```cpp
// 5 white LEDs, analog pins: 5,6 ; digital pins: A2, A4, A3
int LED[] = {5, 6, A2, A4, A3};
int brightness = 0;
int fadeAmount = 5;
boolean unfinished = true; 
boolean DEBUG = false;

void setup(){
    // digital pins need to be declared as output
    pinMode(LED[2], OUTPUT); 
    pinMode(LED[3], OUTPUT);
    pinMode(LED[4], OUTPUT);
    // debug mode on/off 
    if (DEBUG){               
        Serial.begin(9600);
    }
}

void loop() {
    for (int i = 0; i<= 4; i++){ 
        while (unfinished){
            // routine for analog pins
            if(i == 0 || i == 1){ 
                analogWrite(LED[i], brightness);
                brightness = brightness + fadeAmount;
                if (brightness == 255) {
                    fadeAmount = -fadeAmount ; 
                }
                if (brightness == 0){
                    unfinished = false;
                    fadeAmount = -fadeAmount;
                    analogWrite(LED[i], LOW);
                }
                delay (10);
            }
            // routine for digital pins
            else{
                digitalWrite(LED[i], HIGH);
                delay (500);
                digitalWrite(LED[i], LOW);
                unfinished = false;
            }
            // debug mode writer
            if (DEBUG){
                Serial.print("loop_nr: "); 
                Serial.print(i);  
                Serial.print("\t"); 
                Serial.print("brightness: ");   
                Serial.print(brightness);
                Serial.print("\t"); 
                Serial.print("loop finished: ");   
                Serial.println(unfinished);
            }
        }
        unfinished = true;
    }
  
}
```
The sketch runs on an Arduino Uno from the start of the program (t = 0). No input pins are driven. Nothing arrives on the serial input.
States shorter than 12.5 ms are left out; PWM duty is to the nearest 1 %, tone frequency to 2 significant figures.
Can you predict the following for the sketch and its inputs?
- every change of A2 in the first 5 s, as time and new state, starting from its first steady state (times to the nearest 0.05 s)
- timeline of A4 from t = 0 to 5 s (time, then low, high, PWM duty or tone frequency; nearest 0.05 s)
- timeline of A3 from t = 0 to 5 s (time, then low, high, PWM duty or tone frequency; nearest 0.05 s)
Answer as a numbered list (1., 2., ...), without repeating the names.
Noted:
1. 0 s low; 2.05 s high; 2.55 s low
2. 0 s low; 2.55 s high; 3.05 s low
3. 0 s low; 3.05 s high; 3.55 s low
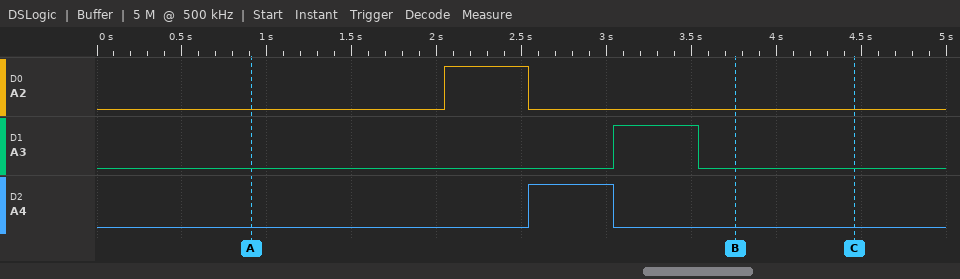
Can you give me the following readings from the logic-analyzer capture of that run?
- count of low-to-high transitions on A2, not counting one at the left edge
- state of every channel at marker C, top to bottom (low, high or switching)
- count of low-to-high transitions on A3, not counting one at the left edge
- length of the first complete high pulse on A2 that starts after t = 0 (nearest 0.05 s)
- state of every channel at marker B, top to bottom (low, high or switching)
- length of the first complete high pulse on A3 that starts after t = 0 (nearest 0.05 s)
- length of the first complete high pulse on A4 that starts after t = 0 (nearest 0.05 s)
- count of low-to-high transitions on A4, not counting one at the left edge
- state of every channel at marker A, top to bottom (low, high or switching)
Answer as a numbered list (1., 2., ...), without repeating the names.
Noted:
1. 1
2. A2 low, A3 low, A4 low
3. 1
4. 0.50 s
5. A2 low, A3 low, A4 low
6. 0.50 s
7. 0.50 s
8. 1
9. A2 low, A3 low, A4 low
